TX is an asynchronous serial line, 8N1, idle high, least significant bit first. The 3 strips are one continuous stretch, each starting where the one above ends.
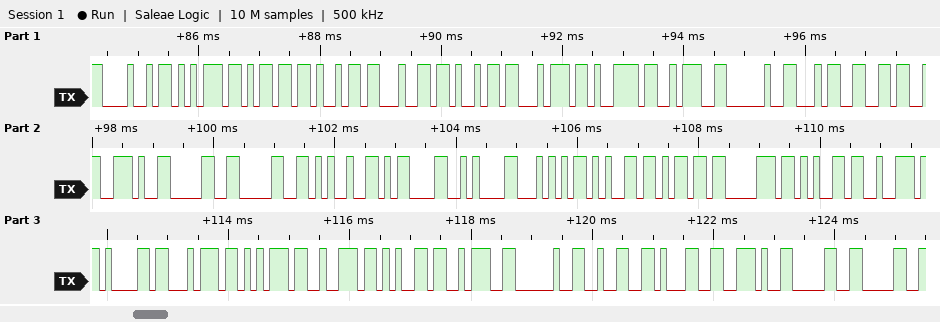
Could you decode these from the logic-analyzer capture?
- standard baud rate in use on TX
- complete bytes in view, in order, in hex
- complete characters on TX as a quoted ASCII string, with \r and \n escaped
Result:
9600 baud
48 75 6D 69 64 69 74 79 3A 20 34 36 2E 30 30 25 0D 0A 54 65 6D 70 65 72 61 74 75 72 65 3A 20 32 31 2E 30 30
"Humidity: 46.00%\r\nTemperature: 21.00"
